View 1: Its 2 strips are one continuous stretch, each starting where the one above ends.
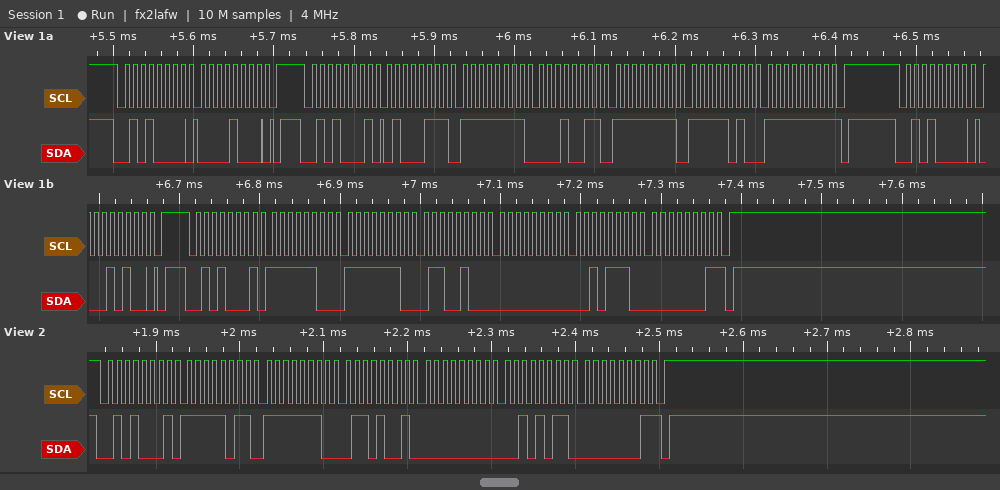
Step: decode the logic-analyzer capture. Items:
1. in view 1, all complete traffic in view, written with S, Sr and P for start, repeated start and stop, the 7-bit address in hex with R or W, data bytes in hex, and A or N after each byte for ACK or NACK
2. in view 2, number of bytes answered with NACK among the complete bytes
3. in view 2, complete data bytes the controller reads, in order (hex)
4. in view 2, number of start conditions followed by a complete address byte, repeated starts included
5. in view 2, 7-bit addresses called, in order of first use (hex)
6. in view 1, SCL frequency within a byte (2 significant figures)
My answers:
S 28W A 08 A P S 28R A 47 A FF A 13 A FF A FA A FF N P S 28W A 14 A P S 28R A FC A FE A 64 A 00 A 2E A 01 N P
1
FB FE 69 00 2B 01
1
0x28
100 kHz
